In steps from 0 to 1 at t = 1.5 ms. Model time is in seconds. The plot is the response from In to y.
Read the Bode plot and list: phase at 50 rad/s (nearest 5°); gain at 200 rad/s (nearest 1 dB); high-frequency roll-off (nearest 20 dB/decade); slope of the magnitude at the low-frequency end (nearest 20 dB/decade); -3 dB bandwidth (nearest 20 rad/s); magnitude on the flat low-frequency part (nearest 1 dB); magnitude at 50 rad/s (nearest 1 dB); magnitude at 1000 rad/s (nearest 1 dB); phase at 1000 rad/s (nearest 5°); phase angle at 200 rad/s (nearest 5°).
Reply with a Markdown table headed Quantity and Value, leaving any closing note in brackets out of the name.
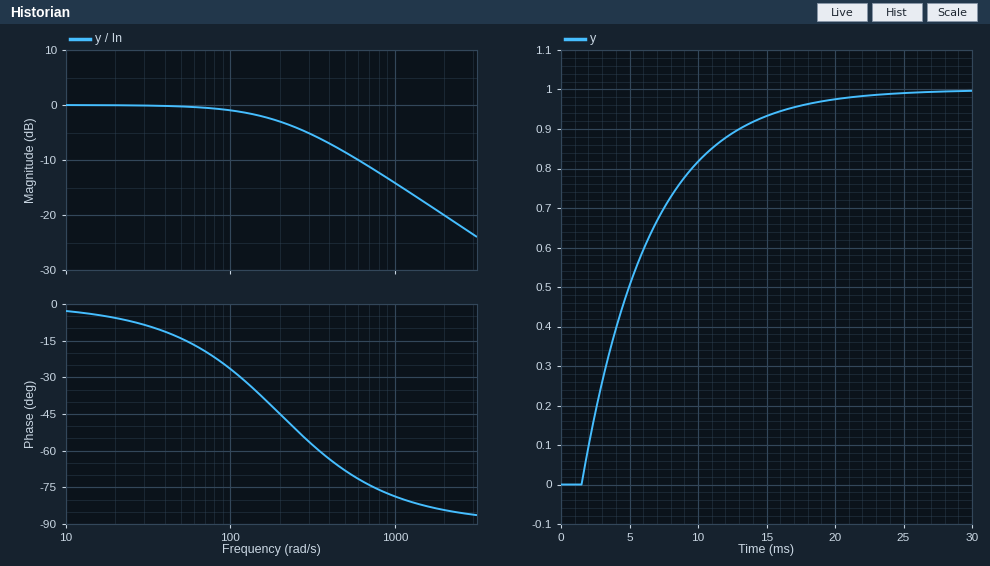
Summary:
| Quantity | Value |
|---|---|
| phase at 50 rad/s | -15° |
| gain at 200 rad/s | -3 dB |
| high-frequency roll-off | -20 dB/decade |
| slope of the magnitude at the low-frequency end | 0 dB/decade |
| -3 dB bandwidth | 200 rad/s |
| magnitude on the flat low-frequency part | 0 dB |
| magnitude at 50 rad/s | 0 dB |
| magnitude at 1000 rad/s | -14 dB |
| phase at 1000 rad/s | -80° |
| phase angle at 200 rad/s | -45° |
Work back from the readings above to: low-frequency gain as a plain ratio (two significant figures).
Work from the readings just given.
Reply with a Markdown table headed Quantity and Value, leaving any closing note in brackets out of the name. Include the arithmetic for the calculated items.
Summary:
| Quantity | Value |
|---|---|
| low-frequency gain as a plain ratio | 10^(0 / 20) = 1.0 |
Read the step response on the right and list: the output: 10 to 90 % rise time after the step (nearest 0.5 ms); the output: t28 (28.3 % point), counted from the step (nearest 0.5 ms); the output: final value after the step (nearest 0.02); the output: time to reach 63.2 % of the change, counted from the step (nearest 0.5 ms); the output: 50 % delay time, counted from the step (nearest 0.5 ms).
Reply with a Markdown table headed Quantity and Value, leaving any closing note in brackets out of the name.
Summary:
| Quantity | Value |
|---|---|
| the output: 10 to 90 % rise time after the step | 11.0 ms |
| the output: t28 (28.3 % point), counted from the step | 1.5 ms |
| the output: final value after the step | 1.00 |
| the output: time to reach 63.2 % of the change, counted from the step | 5.0 ms |
| the output: 50 % delay time, counted from the step | 3.5 ms |
